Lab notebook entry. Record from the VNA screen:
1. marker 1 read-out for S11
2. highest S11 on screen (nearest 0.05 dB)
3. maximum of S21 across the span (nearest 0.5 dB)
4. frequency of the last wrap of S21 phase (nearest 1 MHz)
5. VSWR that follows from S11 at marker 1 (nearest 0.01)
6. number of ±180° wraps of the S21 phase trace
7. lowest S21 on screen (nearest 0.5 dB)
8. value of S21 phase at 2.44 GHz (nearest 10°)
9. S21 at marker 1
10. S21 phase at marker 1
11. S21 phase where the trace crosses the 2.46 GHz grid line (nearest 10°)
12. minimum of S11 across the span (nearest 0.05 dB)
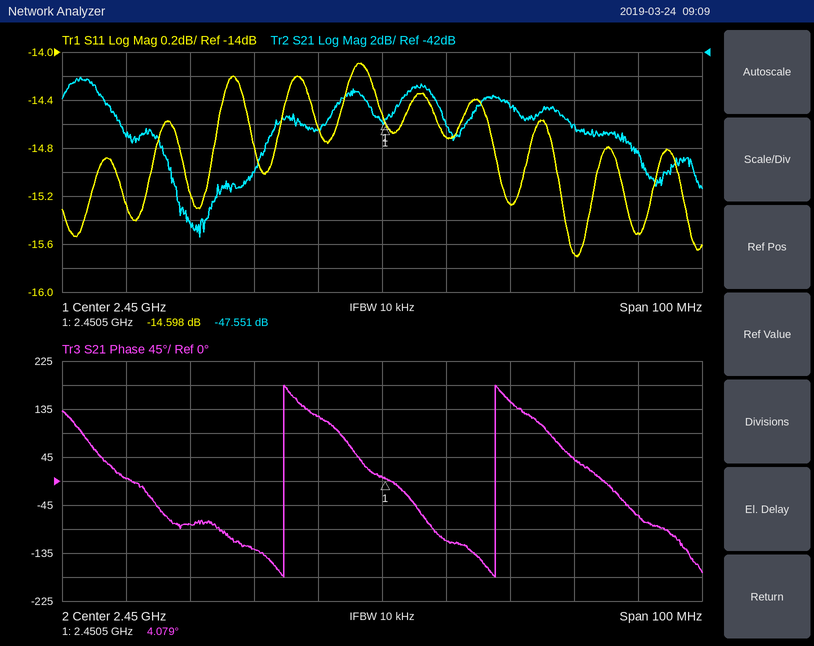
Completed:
-14.598 dB
-14.10 dB
-44.0 dB
2.468 GHz
1.46
2
-57.5 dB
120°
-47.551 dB
4.079°
-110°
-15.70 dB
